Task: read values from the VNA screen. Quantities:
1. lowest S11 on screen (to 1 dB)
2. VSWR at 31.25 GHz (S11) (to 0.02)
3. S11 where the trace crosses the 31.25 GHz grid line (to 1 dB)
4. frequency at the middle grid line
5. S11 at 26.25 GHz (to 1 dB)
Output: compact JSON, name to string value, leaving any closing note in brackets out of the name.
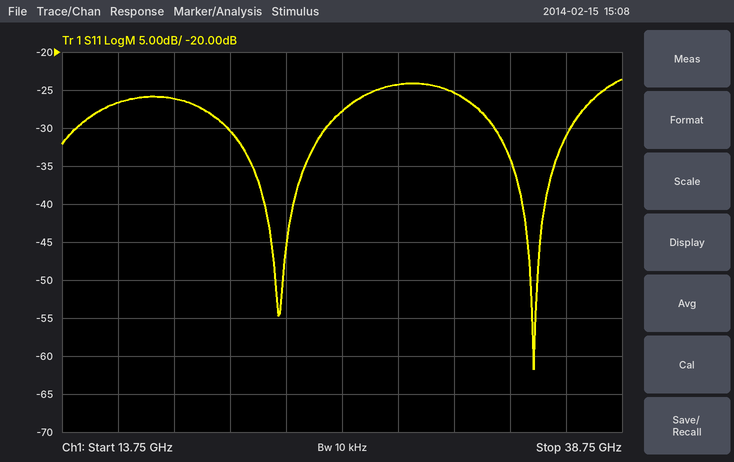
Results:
{"lowest S11 on screen": "-62 dB", "VSWR at 31.25 GHz (S11)": "1.12", "S11 where the trace crosses the 31.25 GHz grid line": "-25 dB", "frequency at the middle grid line": "26.25 GHz", "S11 at 26.25 GHz": "-28 dB"}
